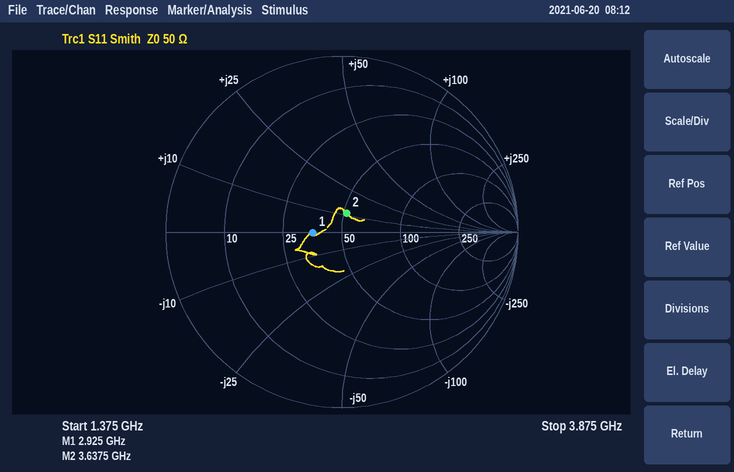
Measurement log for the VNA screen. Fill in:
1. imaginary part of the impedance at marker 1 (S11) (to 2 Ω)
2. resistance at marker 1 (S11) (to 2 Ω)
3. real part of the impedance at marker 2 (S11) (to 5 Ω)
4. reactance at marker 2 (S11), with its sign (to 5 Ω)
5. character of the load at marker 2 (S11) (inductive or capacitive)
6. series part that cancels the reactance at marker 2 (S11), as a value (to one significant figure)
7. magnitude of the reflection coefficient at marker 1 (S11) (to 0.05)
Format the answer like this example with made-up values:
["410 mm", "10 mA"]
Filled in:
["0 Ω", "36 Ω", "50 Ω", "+10 Ω", "inductive", "4 pF", "0.15"]
